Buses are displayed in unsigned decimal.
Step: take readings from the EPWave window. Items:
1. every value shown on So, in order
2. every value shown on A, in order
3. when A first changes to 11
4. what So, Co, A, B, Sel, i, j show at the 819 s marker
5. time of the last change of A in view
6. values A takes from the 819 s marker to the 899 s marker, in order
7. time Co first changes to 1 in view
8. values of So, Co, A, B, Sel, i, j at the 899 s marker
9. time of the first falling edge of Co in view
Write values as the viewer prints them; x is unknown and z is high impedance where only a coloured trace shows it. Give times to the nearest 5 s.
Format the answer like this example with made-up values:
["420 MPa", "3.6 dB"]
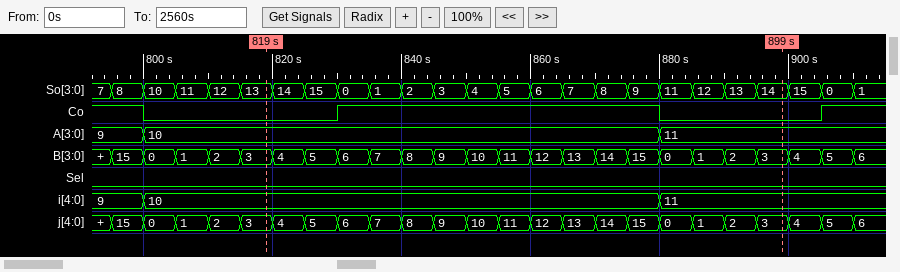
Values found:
["7, 8, 10, 11, 12, 13, 14, 15, 0, 1, 2, 3, 4, 5, 6, 7, 8, 9, 11, 12, 13, 14, 15, 0, 1", "9, 10, 11", "880 s", "So=13, Co=0, A=10, B=3, Sel=0, i=10, j=3", "880 s", "10, 11", "830 s", "So=14, Co=0, A=11, B=3, Sel=0, i=11, j=3", "800 s"]
